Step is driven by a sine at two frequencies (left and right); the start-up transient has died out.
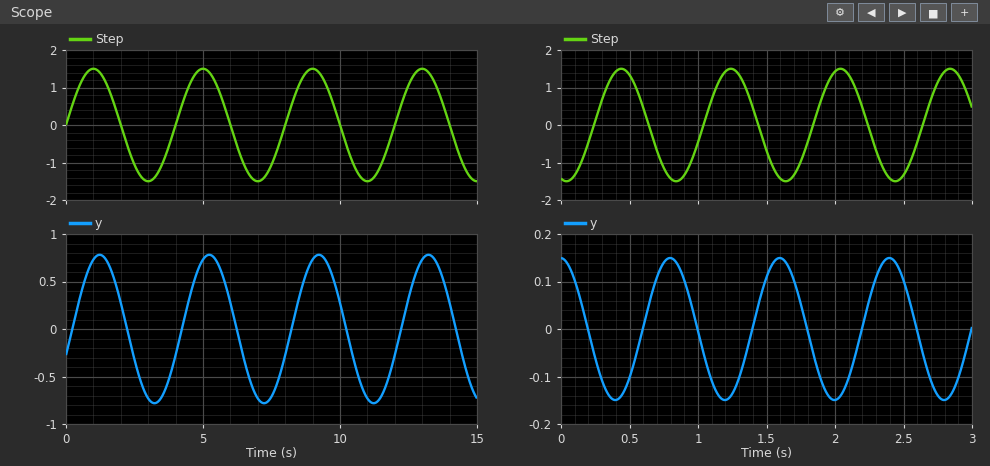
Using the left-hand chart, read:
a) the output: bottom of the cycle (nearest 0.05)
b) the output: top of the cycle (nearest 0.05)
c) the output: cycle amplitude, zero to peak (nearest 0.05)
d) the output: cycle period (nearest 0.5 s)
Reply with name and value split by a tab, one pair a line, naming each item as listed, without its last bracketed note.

the output: bottom of the cycle	-0.80
the output: top of the cycle	0.80
the output: cycle amplitude, zero to peak	0.80
the output: cycle period	4.0 s
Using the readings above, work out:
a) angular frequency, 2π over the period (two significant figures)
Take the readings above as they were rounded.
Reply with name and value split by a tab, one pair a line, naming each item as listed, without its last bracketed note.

angular frequency, 2π over the period	1.6 rad/s
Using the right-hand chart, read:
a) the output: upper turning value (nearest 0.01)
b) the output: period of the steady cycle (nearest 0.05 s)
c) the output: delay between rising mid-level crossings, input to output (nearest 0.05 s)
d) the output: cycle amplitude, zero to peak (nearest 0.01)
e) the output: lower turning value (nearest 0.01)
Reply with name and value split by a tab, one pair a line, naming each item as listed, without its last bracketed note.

the output: upper turning value	0.15
the output: period of the steady cycle	0.80 s
the output: delay between rising mid-level crossings, input to output	0.35 s
the output: cycle amplitude, zero to peak	0.15
the output: lower turning value	-0.15
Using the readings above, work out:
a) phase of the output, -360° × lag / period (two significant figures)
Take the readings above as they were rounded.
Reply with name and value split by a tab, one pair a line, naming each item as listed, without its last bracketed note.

phase of the output, -360° × lag / period	-160°
